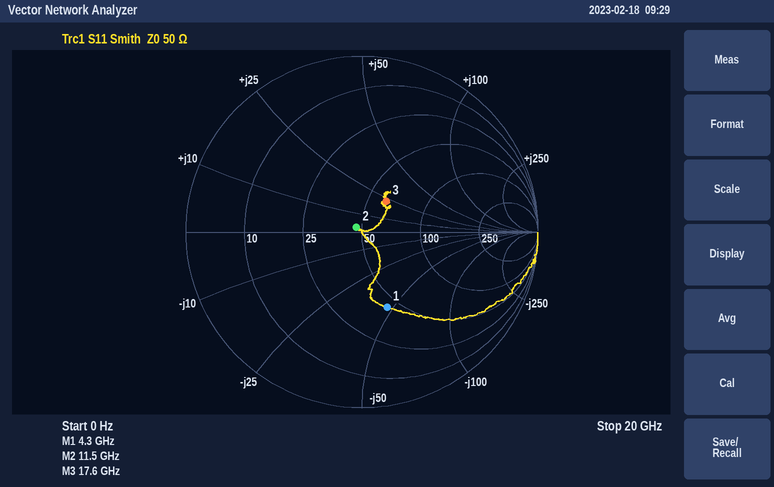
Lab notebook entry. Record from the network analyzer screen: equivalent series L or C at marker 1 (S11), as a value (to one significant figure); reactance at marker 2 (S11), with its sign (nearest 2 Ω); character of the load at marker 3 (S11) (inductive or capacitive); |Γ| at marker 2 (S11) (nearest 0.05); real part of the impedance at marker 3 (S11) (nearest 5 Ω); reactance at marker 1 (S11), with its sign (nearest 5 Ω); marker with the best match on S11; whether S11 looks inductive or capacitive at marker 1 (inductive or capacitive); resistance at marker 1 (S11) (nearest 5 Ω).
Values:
800 fF
+2 Ω
inductive
0.05
60 Ω
-45 Ω
marker 2
capacitive
45 Ω
